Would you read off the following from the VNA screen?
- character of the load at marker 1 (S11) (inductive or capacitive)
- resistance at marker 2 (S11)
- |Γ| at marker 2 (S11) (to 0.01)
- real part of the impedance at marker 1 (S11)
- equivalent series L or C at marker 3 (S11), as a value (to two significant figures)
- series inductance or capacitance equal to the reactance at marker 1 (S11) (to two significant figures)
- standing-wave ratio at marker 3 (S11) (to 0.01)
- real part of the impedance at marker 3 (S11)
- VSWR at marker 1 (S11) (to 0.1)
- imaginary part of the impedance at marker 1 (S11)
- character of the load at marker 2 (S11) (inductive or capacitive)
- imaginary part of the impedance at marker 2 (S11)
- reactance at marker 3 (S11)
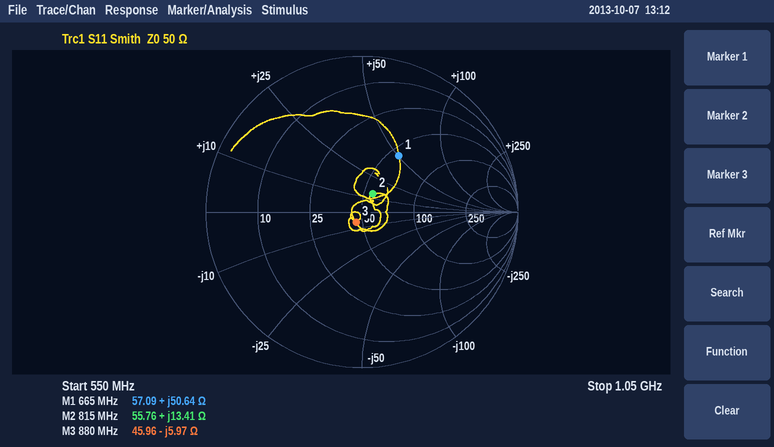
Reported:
inductive
55.76 Ω
0.14
57.09 Ω
30 pF
12 nH
1.16
45.96 Ω
2.5
+50.64 Ω
inductive
+13.41 Ω
-5.97 Ω
